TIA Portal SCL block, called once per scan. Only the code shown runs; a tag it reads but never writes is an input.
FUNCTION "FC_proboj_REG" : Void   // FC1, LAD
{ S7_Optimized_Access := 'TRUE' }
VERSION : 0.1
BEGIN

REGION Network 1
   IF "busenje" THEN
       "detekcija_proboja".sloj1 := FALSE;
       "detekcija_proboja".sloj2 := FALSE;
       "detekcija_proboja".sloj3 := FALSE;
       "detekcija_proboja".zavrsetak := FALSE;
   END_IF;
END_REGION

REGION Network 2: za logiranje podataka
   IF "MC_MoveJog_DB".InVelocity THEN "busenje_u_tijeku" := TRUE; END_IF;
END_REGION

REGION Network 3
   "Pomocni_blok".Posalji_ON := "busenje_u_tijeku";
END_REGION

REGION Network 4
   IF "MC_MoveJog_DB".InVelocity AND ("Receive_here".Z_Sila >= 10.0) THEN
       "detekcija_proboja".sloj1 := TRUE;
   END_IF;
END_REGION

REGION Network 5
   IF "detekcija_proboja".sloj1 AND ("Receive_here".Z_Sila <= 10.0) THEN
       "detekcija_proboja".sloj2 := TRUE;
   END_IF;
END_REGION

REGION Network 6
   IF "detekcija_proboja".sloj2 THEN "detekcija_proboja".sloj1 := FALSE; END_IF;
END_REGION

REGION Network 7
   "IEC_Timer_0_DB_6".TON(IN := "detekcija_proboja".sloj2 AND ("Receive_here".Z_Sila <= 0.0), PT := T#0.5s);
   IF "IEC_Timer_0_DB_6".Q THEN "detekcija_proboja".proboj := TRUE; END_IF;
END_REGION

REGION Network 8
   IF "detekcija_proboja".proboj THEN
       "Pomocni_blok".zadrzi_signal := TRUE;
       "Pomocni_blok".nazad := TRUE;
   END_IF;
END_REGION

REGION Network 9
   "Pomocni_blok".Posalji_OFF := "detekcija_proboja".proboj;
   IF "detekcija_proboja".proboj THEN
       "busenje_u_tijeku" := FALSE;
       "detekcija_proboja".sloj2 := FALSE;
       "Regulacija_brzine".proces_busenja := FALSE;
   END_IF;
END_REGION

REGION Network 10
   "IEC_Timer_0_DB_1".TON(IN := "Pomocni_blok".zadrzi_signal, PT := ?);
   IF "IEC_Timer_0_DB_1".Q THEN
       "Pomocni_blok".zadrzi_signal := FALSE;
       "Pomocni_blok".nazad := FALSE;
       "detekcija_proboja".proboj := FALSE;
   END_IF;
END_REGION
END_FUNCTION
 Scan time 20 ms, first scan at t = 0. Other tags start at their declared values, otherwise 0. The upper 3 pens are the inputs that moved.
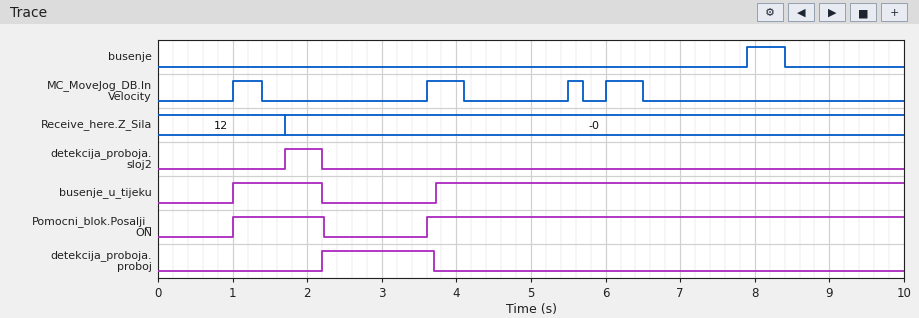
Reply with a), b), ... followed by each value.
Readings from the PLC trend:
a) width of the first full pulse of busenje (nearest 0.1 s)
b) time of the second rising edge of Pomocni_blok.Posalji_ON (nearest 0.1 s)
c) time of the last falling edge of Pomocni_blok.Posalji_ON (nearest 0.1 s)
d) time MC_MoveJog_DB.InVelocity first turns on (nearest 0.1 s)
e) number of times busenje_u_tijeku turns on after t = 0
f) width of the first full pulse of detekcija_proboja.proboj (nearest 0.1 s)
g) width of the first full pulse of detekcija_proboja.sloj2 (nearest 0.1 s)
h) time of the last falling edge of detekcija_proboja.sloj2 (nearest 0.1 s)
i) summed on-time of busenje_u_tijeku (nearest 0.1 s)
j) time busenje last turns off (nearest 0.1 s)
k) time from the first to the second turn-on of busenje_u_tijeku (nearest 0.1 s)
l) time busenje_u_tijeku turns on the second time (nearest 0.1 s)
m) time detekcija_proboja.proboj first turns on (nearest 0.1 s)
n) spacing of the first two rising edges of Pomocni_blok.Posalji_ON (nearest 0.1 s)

a) 0.5 s
b) 3.6 s
c) 2.2 s
d) 1.0 s
e) 2
f) 1.5 s
g) 0.5 s
h) 2.2 s
i) 7.5 s
j) 8.4 s
k) 2.7 s
l) 3.7 s
m) 2.2 s
n) 2.6 s
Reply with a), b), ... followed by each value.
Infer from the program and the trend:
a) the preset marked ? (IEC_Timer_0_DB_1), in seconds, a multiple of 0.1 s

a) 1.5 s
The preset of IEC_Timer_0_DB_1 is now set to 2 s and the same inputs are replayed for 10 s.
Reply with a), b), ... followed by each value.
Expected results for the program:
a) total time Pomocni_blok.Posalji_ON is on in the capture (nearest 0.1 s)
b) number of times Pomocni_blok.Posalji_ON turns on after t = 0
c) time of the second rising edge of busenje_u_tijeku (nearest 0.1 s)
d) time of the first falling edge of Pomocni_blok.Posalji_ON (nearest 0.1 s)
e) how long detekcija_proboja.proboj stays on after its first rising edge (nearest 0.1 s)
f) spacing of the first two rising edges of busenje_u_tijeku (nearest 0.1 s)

a) 6.2 s
b) 3
c) 5.5 s
d) 2.2 s
e) 2.0 s
f) 4.5 s
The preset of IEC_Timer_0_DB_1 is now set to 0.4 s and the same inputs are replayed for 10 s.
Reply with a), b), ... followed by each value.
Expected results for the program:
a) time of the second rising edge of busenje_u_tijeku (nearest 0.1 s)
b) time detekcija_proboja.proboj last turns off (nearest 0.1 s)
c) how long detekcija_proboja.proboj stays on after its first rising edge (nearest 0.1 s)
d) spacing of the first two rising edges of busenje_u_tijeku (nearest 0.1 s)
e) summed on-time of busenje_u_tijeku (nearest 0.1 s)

a) 3.6 s
b) 2.6 s
c) 0.4 s
d) 2.6 s
e) 7.6 s
